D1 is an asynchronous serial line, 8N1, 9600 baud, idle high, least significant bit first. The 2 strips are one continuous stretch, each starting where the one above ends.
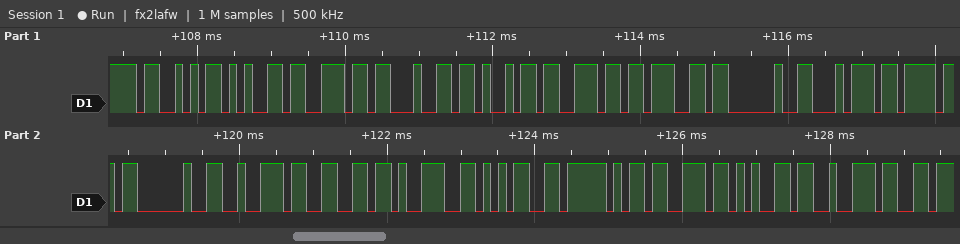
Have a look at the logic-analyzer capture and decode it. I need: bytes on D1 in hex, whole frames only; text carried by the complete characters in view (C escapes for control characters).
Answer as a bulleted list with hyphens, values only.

- 0x53 0x65 0x6E 0x64 0x69 0x6E 0x67 0x20 0x74 0x6F 0x20 0x72 0x66 0x39 0x35 0x5F 0x73 0x65 0x72
- "Sending to rf95_ser"
